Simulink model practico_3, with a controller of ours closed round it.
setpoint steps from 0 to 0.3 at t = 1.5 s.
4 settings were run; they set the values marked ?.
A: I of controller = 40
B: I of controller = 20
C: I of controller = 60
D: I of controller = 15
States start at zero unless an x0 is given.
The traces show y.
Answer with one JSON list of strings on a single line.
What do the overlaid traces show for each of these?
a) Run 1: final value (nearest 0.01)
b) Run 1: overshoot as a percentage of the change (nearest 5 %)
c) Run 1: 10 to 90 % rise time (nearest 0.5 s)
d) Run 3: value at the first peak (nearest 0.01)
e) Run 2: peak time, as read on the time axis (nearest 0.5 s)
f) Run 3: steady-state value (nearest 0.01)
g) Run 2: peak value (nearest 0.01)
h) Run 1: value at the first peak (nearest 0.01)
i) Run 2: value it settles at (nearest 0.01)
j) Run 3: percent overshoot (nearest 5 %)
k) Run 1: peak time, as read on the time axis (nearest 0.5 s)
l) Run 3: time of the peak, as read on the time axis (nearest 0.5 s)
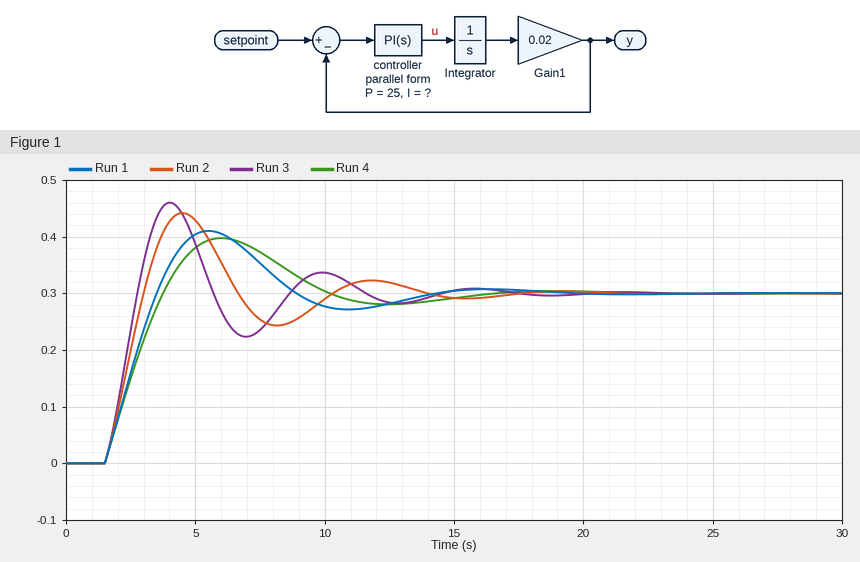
["0.30", "35 %", "1.5 s", "0.46", "4.5 s", "0.30", "0.44", "0.41", "0.30", "55 %", "5.5 s", "4.0 s"]
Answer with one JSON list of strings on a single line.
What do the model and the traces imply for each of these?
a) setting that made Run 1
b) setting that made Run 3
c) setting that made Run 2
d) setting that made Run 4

["B", "C", "A", "D"]
